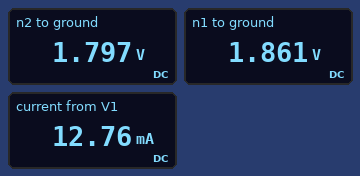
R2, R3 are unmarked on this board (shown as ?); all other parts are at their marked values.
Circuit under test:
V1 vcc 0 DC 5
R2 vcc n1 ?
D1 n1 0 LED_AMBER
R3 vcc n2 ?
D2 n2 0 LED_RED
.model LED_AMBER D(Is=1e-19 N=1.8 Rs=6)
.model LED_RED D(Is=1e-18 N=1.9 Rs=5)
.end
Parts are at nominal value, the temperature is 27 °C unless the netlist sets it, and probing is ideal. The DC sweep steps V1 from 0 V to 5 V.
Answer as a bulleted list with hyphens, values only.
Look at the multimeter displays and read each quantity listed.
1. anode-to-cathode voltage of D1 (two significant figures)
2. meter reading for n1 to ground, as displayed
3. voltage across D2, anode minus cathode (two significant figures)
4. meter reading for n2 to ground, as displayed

- 1.9 V
- 1.861 V
- 1.8 V
- 1.797 V
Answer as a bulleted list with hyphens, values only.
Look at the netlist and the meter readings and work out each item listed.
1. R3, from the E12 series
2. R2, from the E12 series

- 680 Ω
- 390 Ω
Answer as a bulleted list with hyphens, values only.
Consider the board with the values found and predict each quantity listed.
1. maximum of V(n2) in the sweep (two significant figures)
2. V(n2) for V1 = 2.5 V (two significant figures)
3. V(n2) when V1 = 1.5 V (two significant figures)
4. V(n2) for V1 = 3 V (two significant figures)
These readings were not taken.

- 1.8 V
- 1.7 V
- 1.5 V
- 1.7 V
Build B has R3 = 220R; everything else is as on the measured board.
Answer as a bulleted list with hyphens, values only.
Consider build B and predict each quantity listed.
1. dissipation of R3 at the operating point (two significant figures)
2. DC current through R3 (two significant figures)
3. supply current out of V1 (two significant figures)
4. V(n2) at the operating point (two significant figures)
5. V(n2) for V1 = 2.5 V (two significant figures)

- 44 mW
- 14 mA
- 22 mA
- 1.9 V
- 1.8 V
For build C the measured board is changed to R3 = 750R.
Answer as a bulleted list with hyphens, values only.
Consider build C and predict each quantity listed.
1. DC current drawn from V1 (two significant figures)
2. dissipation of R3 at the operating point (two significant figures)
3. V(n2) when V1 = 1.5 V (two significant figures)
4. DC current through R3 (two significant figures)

- 12 mA
- 14 mW
- 1.5 V
- 4.3 mA
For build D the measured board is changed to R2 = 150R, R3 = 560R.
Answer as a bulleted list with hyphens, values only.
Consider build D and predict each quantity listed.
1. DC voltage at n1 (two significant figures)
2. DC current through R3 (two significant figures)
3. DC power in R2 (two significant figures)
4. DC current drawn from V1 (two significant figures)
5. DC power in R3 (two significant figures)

- 2.0 V
- 5.7 mA
- 61 mW
- 26 mA
- 18 mW
